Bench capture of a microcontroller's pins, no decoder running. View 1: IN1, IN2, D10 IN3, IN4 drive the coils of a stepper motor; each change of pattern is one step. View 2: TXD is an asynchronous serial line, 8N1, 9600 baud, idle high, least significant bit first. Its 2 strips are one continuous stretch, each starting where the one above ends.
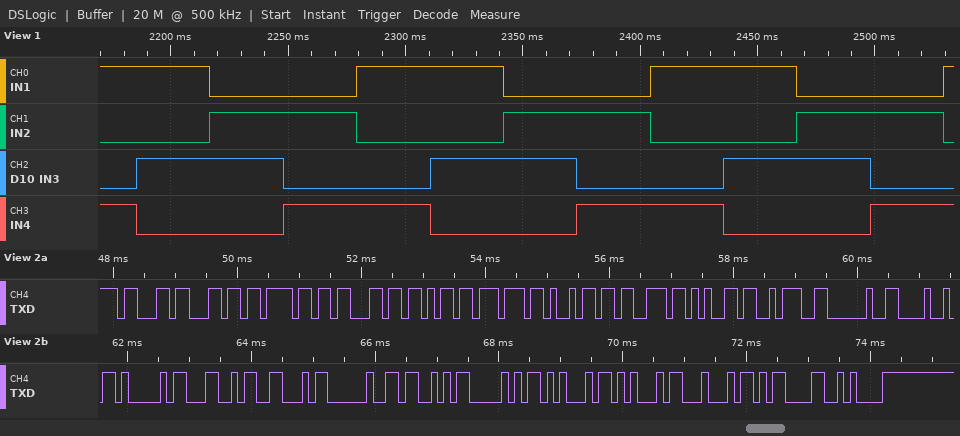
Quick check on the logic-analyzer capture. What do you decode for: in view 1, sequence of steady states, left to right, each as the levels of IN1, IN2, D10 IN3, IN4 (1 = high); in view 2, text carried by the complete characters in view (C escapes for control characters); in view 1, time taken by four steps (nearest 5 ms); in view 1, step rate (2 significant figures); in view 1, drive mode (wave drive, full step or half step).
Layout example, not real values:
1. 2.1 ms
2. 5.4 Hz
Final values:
1. 1001 1010 0110 0101 1001 1010 0110 0101 1001 1010 0110 0101 1001
2. "clockwise: HALF SPEED\r\n"
3. 125 ms
4. 32 steps/s
5. full step
